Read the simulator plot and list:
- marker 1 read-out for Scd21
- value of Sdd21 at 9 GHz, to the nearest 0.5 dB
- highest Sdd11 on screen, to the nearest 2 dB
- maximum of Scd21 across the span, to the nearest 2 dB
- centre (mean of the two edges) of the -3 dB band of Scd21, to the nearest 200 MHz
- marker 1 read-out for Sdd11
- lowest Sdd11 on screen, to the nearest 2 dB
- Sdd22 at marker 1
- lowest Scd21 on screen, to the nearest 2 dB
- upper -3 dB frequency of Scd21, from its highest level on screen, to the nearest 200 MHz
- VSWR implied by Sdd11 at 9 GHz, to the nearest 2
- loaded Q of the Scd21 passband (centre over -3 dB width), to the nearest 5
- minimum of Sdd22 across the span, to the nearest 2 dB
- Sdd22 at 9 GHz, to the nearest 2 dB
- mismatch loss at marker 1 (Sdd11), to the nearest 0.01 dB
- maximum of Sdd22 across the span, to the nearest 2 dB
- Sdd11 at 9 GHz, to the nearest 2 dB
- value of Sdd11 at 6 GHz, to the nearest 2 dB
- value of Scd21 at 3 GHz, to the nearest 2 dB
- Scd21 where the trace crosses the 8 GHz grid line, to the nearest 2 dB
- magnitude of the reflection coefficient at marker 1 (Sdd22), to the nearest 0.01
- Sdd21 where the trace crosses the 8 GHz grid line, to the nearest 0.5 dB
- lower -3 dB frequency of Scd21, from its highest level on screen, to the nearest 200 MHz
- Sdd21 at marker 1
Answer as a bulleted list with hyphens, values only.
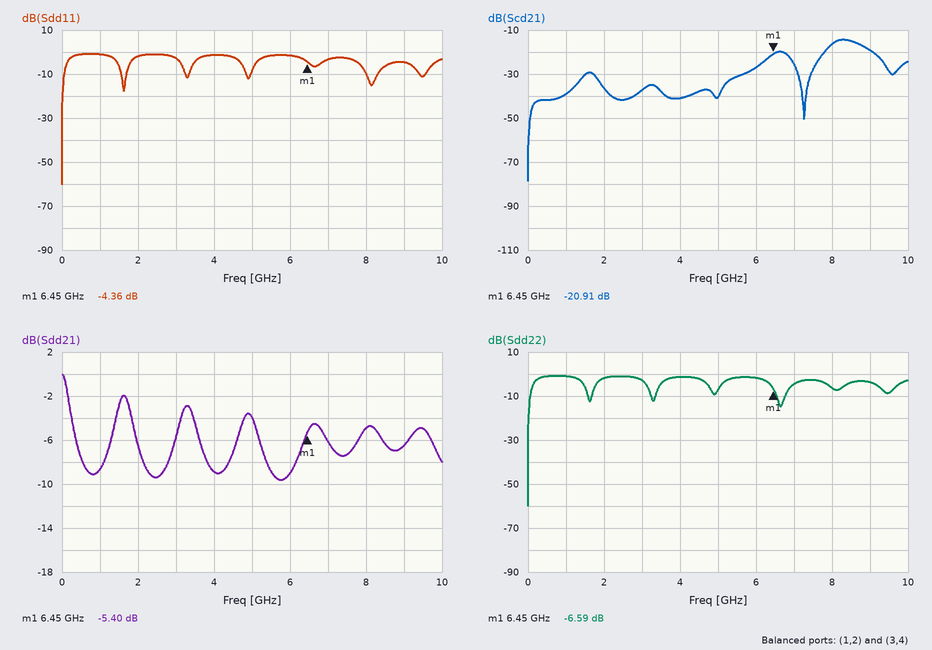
- -20.91 dB
- -6.5 dB
- 0 dB
- -14 dB
- 8.4 GHz
- -4.36 dB
- -60 dB
- -6.59 dB
- -78 dB
- 8.8 GHz
- 4
- 10
- -60 dB
- -4 dB
- 1.98 dB
- 0 dB
- -4 dB
- -2 dB
- -38 dB
- -16 dB
- 0.47
- -5.0 dB
- 8.0 GHz
- -5.40 dB
